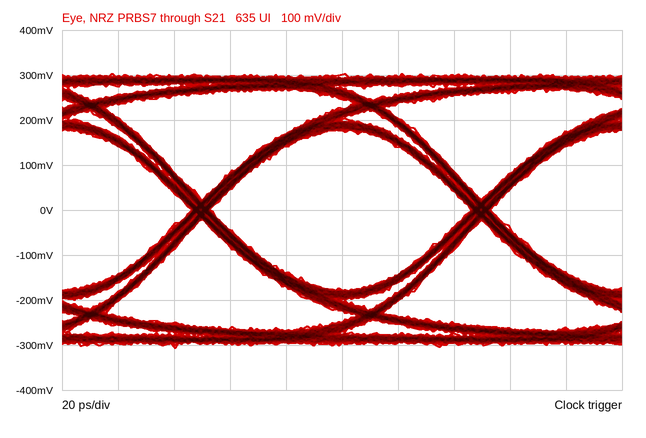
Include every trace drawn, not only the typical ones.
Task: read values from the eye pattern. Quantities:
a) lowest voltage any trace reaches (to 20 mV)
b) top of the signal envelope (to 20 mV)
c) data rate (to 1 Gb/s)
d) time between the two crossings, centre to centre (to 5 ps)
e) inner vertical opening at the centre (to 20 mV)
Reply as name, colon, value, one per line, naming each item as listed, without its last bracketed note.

lowest voltage any trace reaches: -300 mV
top of the signal envelope: 300 mV
data rate: 10 Gb/s
time between the two crossings, centre to centre: 100 ps
inner vertical opening at the centre: 360 mV
